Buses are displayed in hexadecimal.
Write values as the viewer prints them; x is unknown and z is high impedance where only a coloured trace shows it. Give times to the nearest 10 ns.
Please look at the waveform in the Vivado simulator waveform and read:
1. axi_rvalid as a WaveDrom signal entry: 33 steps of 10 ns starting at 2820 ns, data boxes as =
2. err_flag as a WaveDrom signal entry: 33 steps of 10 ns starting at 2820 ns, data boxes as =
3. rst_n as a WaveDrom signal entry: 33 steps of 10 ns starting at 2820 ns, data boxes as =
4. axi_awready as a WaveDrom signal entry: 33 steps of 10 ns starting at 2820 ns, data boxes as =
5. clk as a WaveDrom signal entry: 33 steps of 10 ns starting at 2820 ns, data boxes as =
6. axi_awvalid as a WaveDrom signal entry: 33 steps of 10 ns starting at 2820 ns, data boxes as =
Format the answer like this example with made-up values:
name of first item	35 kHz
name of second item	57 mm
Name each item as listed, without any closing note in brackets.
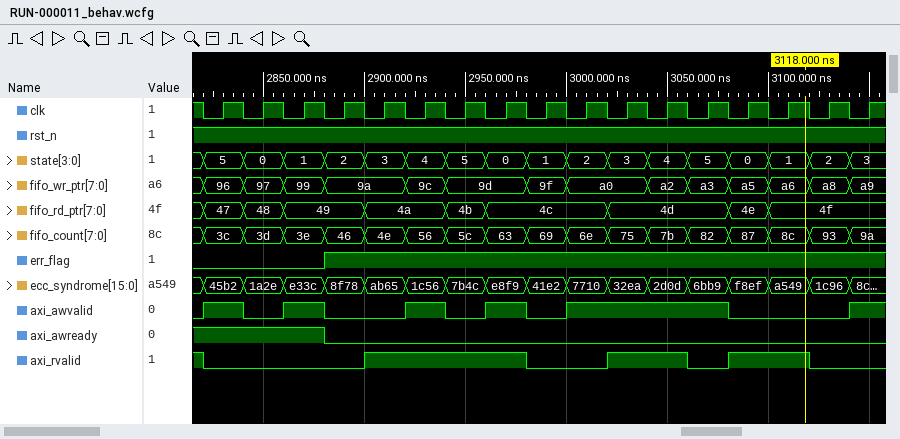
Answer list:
axi_rvalid as a WaveDrom signal entry: 33 steps of 10 ns starting at 2820 ns, data boxes as =	{name: 'axi_rvalid', wave: '0.......1.......0...1...0.1...0..'}
err_flag as a WaveDrom signal entry: 33 steps of 10 ns starting at 2820 ns, data boxes as =	{name: 'err_flag', wave: '0.....1..........................'}
rst_n as a WaveDrom signal entry: 33 steps of 10 ns starting at 2820 ns, data boxes as =	{name: 'rst_n', wave: '1................................'}
axi_awready as a WaveDrom signal entry: 33 steps of 10 ns starting at 2820 ns, data boxes as =	{name: 'axi_awready', wave: '1.....0..........................'}
clk as a WaveDrom signal entry: 33 steps of 10 ns starting at 2820 ns, data boxes as =	{name: 'clk', wave: '010101010101010101010101010101010'}
axi_awvalid as a WaveDrom signal entry: 33 steps of 10 ns starting at 2820 ns, data boxes as =	{name: 'axi_awvalid', wave: '1.0.1.0...1.0.1.0.1.......0.....1'}
